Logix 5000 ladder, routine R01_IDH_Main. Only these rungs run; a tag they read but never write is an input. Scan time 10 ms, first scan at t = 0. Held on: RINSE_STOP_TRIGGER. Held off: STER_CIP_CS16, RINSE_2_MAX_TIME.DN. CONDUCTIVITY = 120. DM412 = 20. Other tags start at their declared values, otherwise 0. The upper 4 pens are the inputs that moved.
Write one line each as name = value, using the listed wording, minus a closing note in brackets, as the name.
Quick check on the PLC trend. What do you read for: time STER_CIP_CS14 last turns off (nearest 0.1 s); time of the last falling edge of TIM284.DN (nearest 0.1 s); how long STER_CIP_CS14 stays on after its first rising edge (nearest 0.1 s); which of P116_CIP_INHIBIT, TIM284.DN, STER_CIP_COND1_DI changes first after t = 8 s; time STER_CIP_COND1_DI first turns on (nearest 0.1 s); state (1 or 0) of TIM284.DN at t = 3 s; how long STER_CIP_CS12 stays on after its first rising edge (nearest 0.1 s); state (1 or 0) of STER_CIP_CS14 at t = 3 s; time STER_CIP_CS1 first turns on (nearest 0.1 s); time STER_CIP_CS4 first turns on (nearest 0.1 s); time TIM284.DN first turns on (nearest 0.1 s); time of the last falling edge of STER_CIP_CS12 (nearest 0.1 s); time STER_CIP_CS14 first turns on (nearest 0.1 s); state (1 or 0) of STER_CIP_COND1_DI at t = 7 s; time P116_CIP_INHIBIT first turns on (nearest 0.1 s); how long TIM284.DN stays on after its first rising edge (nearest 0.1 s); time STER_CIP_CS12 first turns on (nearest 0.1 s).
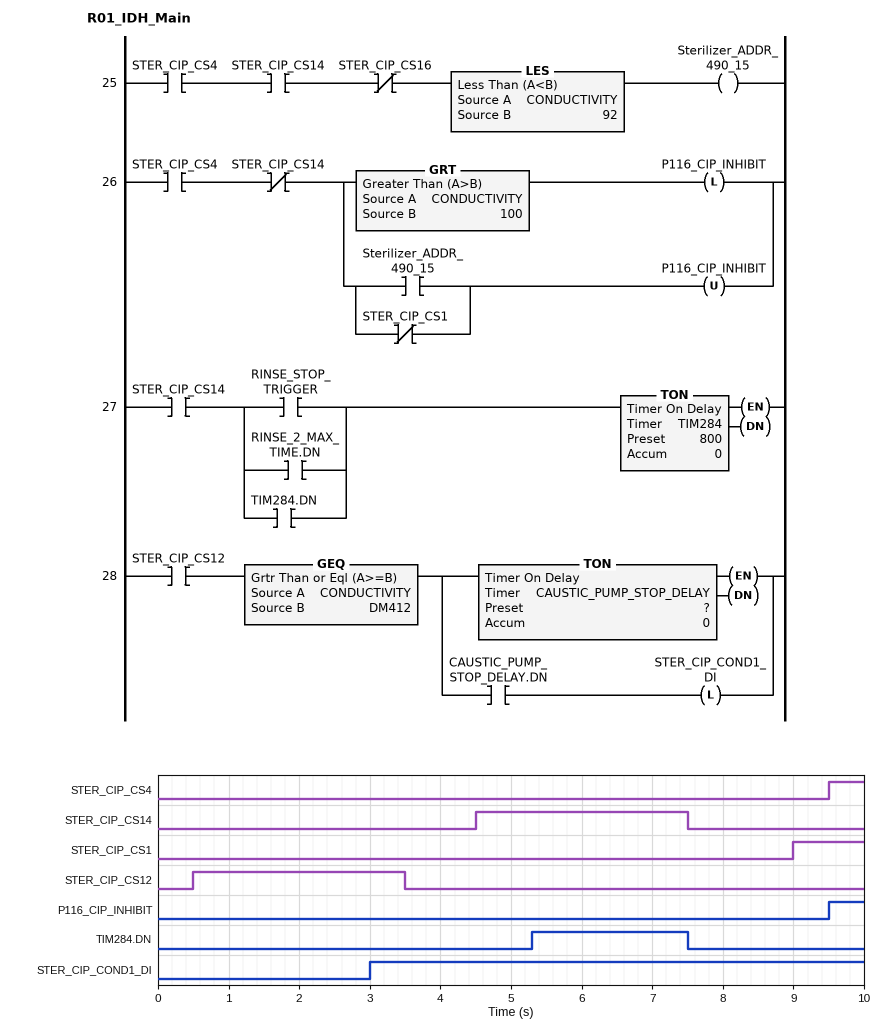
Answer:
time STER_CIP_CS14 last turns off = 7.5 s
time of the last falling edge of TIM284.DN = 7.5 s
how long STER_CIP_CS14 stays on after its first rising edge = 3.0 s
which of P116_CIP_INHIBIT, TIM284.DN, STER_CIP_COND1_DI changes first after t = 8 s = P116_CIP_INHIBIT
time STER_CIP_COND1_DI first turns on = 3.0 s
state (1 or 0) of TIM284.DN at t = 3 s = 0
how long STER_CIP_CS12 stays on after its first rising edge = 3.0 s
state (1 or 0) of STER_CIP_CS14 at t = 3 s = 0
time STER_CIP_CS1 first turns on = 9.0 s
time STER_CIP_CS4 first turns on = 9.5 s
time TIM284.DN first turns on = 5.3 s
time of the last falling edge of STER_CIP_CS12 = 3.5 s
time STER_CIP_CS14 first turns on = 4.5 s
state (1 or 0) of STER_CIP_COND1_DI at t = 7 s = 1
time P116_CIP_INHIBIT first turns on = 9.5 s
how long TIM284.DN stays on after its first rising edge = 2.2 s
time STER_CIP_CS12 first turns on = 0.5 s
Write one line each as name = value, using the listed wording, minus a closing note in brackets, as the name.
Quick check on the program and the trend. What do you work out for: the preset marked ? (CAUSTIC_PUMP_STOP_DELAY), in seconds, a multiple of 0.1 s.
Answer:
the preset marked ? (CAUSTIC_PUMP_STOP_DELAY), in seconds, a multiple of 0.1 s = 2.5 s
